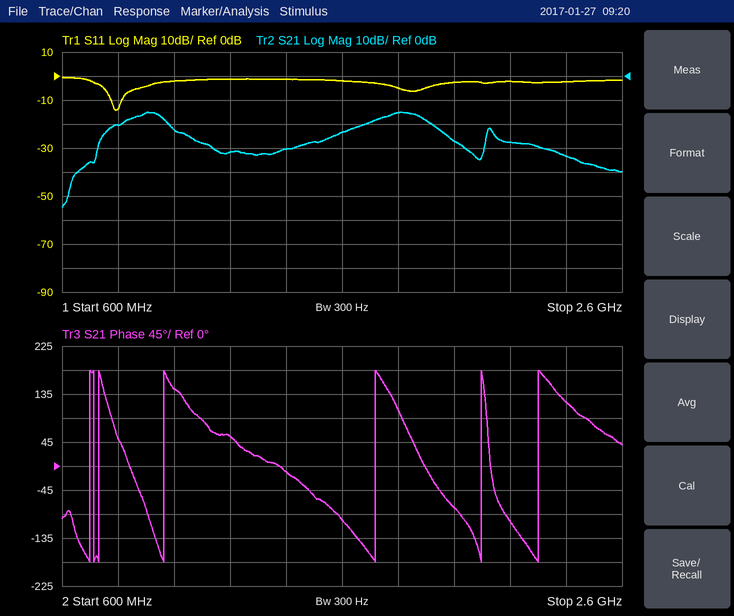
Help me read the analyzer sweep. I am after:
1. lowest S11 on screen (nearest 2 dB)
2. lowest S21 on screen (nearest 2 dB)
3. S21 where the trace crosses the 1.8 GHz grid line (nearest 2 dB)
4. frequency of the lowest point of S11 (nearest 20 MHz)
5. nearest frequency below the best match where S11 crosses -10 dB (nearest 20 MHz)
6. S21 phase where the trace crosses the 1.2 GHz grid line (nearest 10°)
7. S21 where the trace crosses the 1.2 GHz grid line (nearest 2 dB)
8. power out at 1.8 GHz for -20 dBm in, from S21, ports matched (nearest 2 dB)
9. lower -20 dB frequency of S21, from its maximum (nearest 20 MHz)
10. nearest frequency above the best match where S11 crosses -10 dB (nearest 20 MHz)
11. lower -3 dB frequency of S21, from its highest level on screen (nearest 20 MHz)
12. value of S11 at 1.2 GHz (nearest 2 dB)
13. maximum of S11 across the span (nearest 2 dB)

-14 dB
-54 dB
-16 dB
800 MHz
780 MHz
60°
-32 dB
-36 dBm
720 MHz
820 MHz
840 MHz
-2 dB
0 dB
